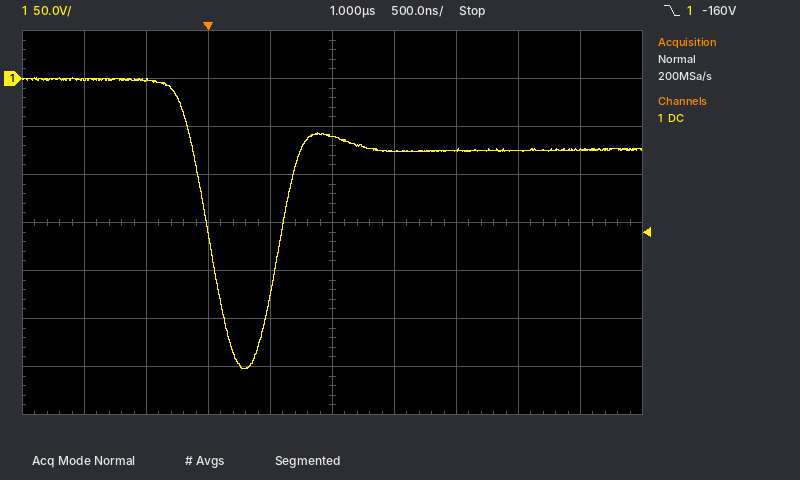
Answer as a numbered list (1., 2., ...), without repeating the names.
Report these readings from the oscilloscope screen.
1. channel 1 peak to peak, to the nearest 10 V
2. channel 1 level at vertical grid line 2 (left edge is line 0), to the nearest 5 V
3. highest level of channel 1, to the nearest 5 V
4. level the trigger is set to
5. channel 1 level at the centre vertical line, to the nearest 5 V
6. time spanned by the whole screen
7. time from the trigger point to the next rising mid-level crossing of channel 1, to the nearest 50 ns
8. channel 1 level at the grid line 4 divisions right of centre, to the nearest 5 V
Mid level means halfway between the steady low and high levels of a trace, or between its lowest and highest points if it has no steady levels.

1. 300 V
2. 0 V
3. 0 V
4. -160 V
5. -60 V
6. 5 µs
7. 600 ns
8. -75 V
